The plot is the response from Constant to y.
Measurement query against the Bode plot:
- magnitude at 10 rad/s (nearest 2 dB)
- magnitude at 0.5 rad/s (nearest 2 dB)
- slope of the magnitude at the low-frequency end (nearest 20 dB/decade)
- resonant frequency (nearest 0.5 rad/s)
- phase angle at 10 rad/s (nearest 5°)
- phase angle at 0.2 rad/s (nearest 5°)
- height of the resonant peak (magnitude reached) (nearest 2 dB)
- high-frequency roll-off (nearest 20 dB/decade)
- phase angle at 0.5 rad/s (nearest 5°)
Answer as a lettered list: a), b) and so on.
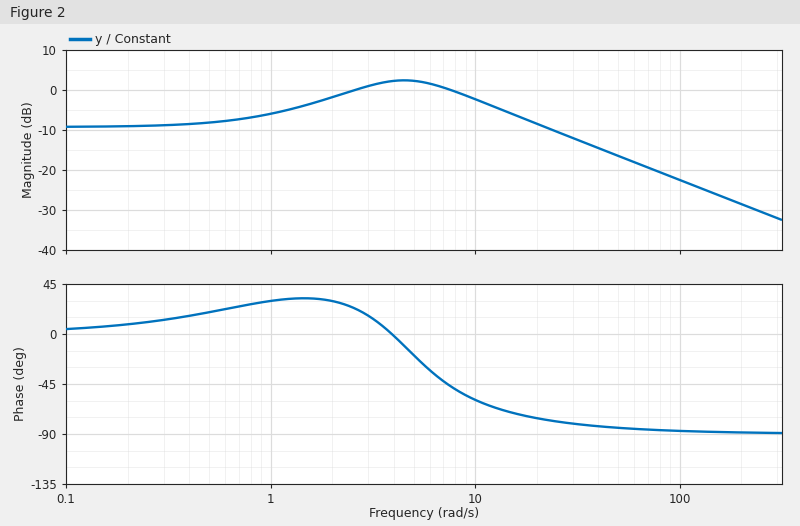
a) -2 dB
b) -8 dB
c) 0 dB/decade
d) 4.5 rad/s
e) -60°
f) 10°
g) 2 dB
h) -20 dB/decade
i) 20°
